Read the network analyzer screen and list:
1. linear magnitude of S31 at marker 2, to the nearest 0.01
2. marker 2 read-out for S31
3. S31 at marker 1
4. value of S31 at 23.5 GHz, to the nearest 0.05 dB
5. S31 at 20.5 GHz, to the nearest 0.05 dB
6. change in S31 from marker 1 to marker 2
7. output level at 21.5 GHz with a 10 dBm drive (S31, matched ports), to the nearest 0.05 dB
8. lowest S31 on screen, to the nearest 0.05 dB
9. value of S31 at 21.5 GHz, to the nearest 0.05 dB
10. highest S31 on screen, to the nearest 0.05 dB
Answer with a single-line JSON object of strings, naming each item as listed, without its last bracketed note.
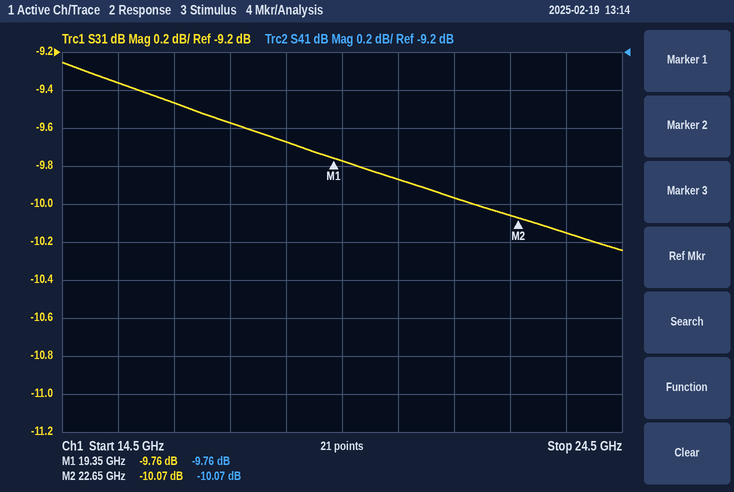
{"linear magnitude of S31 at marker 2, to the nearest 0.01": "0.31", "marker 2 read-out for S31": "-10.07 dB", "S31 at marker 1": "-9.76 dB", "value of S31 at 23.5 GHz, to the nearest 0.05 dB": "-10.15 dB", "S31 at 20.5 GHz, to the nearest 0.05 dB": "-9.85 dB", "change in S31 from marker 1 to marker 2": "-0.31 dB", "output level at 21.5 GHz with a 10 dBm drive (S31, matched ports), to the nearest 0.05 dB": "0.05 dBm", "lowest S31 on screen, to the nearest 0.05 dB": "-10.25 dB", "value of S31 at 21.5 GHz, to the nearest 0.05 dB": "-9.95 dB", "highest S31 on screen, to the nearest 0.05 dB": "-9.25 dB"}
